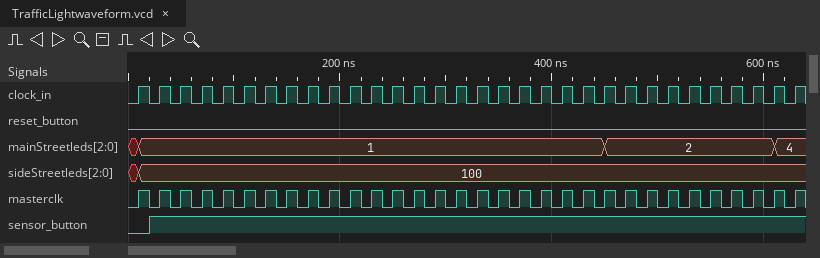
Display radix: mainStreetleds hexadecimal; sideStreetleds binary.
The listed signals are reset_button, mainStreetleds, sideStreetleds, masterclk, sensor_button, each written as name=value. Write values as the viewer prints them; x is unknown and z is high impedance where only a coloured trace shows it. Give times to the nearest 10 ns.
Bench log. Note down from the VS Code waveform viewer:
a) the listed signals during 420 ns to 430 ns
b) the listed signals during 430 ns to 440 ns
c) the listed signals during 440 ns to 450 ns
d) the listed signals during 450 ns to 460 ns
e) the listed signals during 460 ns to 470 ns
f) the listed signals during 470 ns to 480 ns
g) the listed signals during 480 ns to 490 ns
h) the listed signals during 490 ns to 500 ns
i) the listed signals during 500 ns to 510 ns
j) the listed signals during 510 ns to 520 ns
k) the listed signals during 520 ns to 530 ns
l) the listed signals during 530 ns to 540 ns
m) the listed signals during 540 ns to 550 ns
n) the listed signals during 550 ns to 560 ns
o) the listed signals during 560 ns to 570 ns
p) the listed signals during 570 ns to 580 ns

reset_button=0, mainStreetleds=1, sideStreetleds=100, masterclk=0, sensor_button=1
reset_button=0, mainStreetleds=1, sideStreetleds=100, masterclk=1, sensor_button=1
reset_button=0, mainStreetleds=1, sideStreetleds=100, masterclk=0, sensor_button=1
reset_button=0, mainStreetleds=2, sideStreetleds=100, masterclk=1, sensor_button=1
reset_button=0, mainStreetleds=2, sideStreetleds=100, masterclk=0, sensor_button=1
reset_button=0, mainStreetleds=2, sideStreetleds=100, masterclk=1, sensor_button=1
reset_button=0, mainStreetleds=2, sideStreetleds=100, masterclk=0, sensor_button=1
reset_button=0, mainStreetleds=2, sideStreetleds=100, masterclk=1, sensor_button=1
reset_button=0, mainStreetleds=2, sideStreetleds=100, masterclk=0, sensor_button=1
reset_button=0, mainStreetleds=2, sideStreetleds=100, masterclk=1, sensor_button=1
reset_button=0, mainStreetleds=2, sideStreetleds=100, masterclk=0, sensor_button=1
reset_button=0, mainStreetleds=2, sideStreetleds=100, masterclk=1, sensor_button=1
reset_button=0, mainStreetleds=2, sideStreetleds=100, masterclk=0, sensor_button=1
reset_button=0, mainStreetleds=2, sideStreetleds=100, masterclk=1, sensor_button=1
reset_button=0, mainStreetleds=2, sideStreetleds=100, masterclk=0, sensor_button=1
reset_button=0, mainStreetleds=2, sideStreetleds=100, masterclk=1, sensor_button=1
